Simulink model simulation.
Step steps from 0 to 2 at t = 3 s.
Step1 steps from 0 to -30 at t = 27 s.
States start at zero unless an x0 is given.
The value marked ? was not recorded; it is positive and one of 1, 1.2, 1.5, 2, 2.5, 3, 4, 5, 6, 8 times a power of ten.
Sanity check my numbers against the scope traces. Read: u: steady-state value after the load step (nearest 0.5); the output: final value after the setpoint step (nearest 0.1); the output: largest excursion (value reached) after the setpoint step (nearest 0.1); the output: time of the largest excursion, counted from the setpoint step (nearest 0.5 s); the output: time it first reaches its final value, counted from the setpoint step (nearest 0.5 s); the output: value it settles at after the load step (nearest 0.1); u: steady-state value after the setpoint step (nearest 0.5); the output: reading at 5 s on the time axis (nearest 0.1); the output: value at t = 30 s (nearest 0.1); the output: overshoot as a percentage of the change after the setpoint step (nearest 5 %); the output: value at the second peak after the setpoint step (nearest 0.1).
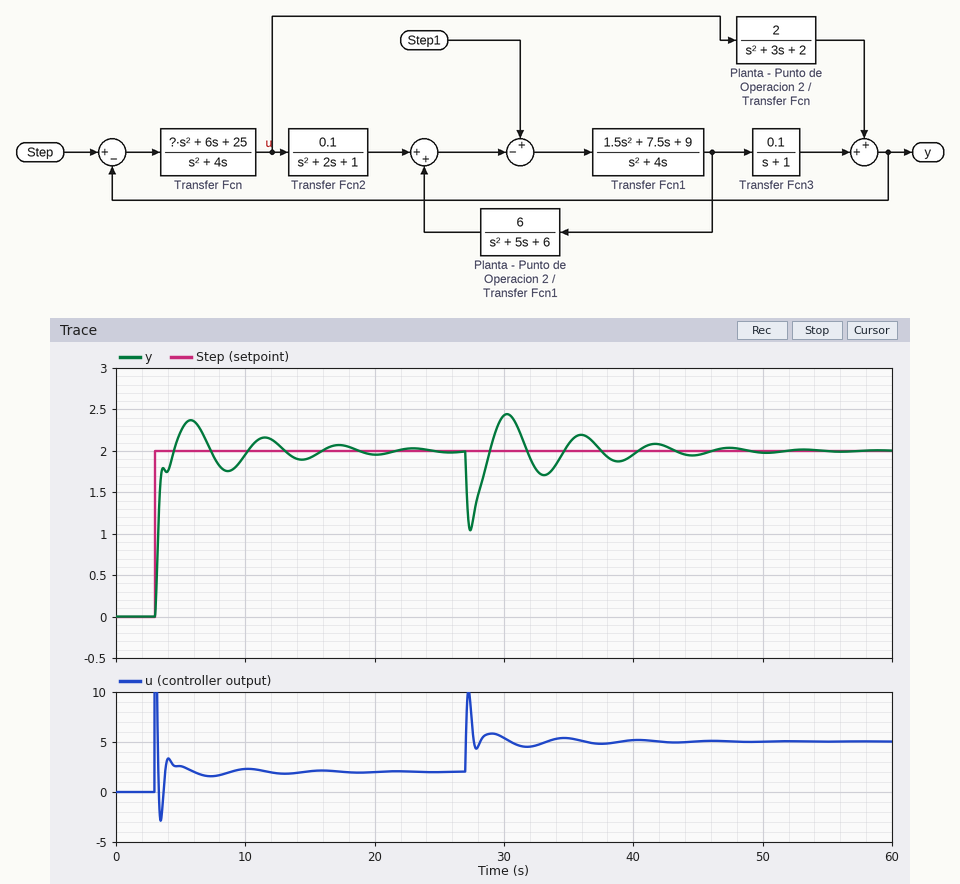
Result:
5.0
2.0
2.4
3.0 s
1.5 s
2.0
2.0
2.2
2.4
20 %
2.2
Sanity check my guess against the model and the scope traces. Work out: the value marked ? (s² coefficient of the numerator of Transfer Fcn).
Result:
15
